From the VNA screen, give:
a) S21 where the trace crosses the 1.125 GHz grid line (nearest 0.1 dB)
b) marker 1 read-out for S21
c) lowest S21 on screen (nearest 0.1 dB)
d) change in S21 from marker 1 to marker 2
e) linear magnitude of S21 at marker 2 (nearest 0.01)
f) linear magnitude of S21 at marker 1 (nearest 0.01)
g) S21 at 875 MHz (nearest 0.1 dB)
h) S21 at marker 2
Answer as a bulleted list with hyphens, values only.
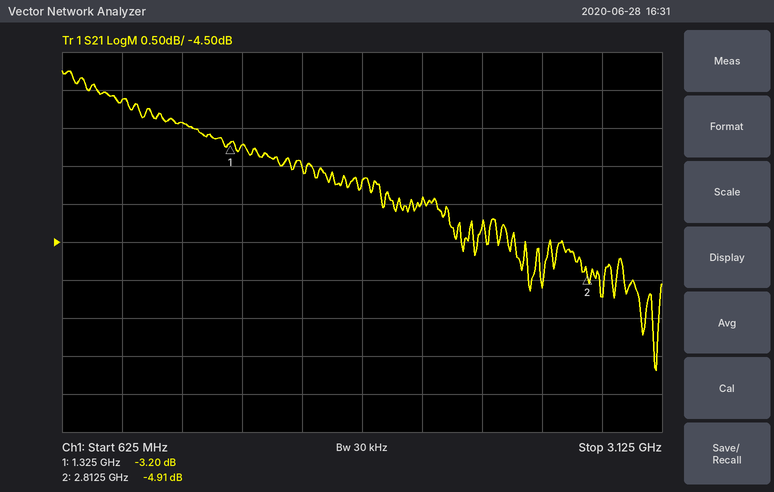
- -2.9 dB
- -3.20 dB
- -6.2 dB
- -1.71 dB
- 0.57
- 0.69
- -2.6 dB
- -4.91 dB
